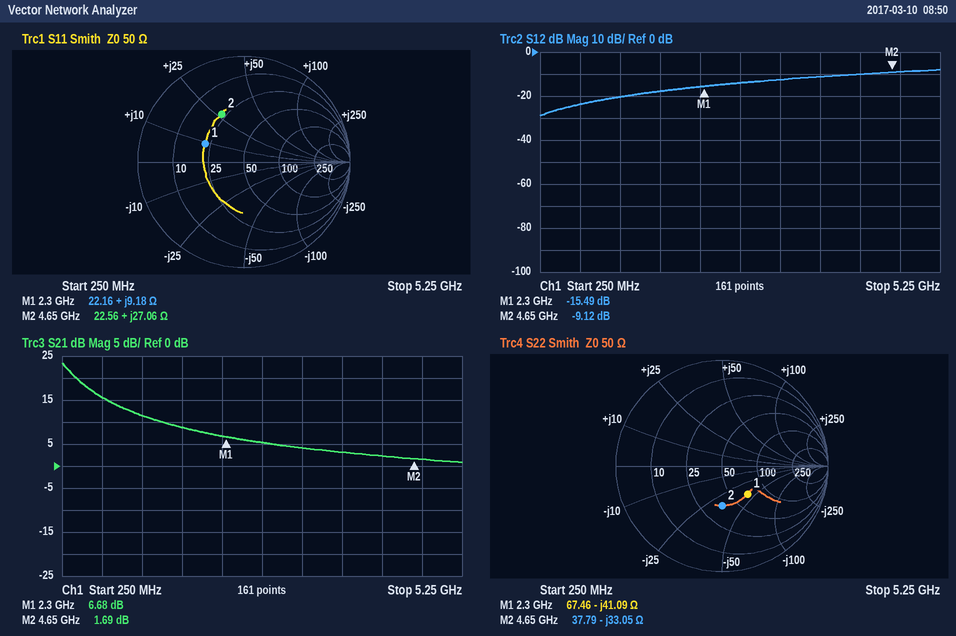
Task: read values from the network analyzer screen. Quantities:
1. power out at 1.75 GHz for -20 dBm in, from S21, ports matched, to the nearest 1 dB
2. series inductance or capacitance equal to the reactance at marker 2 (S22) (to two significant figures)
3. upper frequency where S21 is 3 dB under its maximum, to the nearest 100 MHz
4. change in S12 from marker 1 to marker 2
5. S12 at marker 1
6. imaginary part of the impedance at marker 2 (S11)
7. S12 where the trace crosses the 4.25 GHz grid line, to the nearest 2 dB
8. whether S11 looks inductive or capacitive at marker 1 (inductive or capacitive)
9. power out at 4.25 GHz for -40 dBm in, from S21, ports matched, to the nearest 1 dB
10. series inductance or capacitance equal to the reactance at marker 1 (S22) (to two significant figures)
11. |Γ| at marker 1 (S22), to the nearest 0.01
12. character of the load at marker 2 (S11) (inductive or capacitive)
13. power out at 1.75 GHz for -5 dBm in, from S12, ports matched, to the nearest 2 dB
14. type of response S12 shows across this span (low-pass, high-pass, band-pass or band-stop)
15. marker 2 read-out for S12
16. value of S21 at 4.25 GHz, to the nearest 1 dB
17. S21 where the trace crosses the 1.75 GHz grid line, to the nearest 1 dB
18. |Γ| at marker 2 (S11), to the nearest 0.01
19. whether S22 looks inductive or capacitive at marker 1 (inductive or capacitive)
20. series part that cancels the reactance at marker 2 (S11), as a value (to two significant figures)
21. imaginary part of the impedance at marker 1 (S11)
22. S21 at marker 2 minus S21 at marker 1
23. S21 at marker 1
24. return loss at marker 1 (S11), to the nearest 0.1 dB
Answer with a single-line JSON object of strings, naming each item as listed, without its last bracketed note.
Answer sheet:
{"power out at 1.75 GHz for -20 dBm in, from S21, ports matched, to the nearest 1 dB": "-11 dBm", "series inductance or capacitance equal to the reactance at marker 2 (S22)": "1.0 pF", "upper frequency where S21 is 3 dB under its maximum, to the nearest 100 MHz": "400 MHz", "change in S12 from marker 1 to marker 2": "6.37 dB", "S12 at marker 1": "-15.49 dB", "imaginary part of the impedance at marker 2": "+27.06 Ω", "S12 where the trace crosses the 4.25 GHz grid line, to the nearest 2 dB": "-10 dB", "whether S11 looks inductive or capacitive at marker 1": "inductive", "power out at 4.25 GHz for -40 dBm in, from S21, ports matched, to the nearest 1 dB": "-38 dBm", "series inductance or capacitance equal to the reactance at marker 1 (S22)": "1.7 pF", "|Γ| at marker 1 (S22), to the nearest 0.01": "0.36", "character of the load at marker 2 (S11)": "inductive", "power out at 1.75 GHz for -5 dBm in, from S12, ports matched, to the nearest 2 dB": "-22 dBm", "type of response S12 shows across this span": "high-pass", "marker 2 read-out for S12": "-9.12 dB", "value of S21 at 4.25 GHz, to the nearest 1 dB": "2 dB", "S21 where the trace crosses the 1.75 GHz grid line, to the nearest 1 dB": "9 dB", "|Γ| at marker 2 (S11), to the nearest 0.01": "0.50", "whether S22 looks inductive or capacitive at marker 1": "capacitive", "series part that cancels the reactance at marker 2 (S11), as a value": "1.3 pF", "imaginary part of the impedance at marker 1": "+9.18 Ω", "S21 at marker 2 minus S21 at marker 1": "-4.99 dB", "S21 at marker 1": "6.68 dB", "return loss at marker 1 (S11), to the nearest 0.1 dB": "7.9 dB"}
